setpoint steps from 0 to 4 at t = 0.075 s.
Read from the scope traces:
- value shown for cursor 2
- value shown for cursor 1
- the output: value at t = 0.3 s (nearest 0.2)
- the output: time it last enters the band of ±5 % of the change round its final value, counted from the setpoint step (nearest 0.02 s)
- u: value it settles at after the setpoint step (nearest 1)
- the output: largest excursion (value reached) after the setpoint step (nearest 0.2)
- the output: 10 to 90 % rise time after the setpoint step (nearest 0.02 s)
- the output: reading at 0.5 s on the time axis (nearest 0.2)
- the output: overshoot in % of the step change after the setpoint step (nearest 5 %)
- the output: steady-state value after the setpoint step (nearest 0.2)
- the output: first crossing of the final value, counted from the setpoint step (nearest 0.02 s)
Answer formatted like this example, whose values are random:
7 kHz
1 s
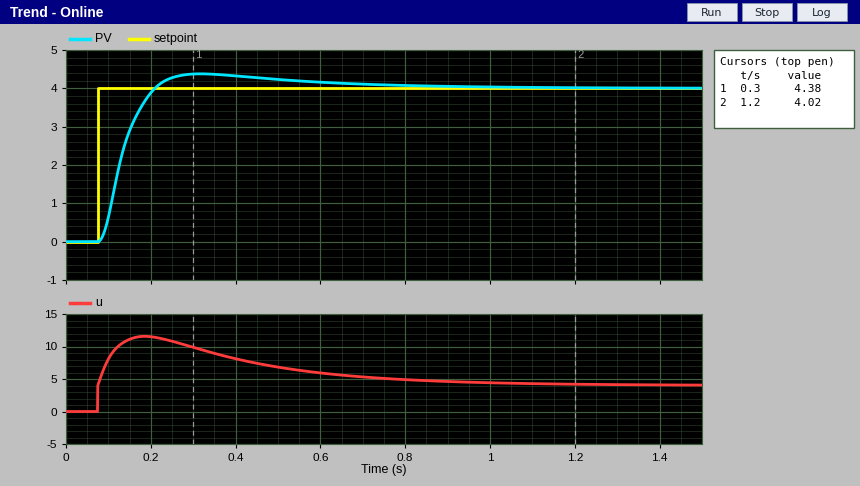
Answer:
4.02
4.38
4.4
0.46 s
4
4.4
0.08 s
4.2
10 %
4.0
0.14 s
